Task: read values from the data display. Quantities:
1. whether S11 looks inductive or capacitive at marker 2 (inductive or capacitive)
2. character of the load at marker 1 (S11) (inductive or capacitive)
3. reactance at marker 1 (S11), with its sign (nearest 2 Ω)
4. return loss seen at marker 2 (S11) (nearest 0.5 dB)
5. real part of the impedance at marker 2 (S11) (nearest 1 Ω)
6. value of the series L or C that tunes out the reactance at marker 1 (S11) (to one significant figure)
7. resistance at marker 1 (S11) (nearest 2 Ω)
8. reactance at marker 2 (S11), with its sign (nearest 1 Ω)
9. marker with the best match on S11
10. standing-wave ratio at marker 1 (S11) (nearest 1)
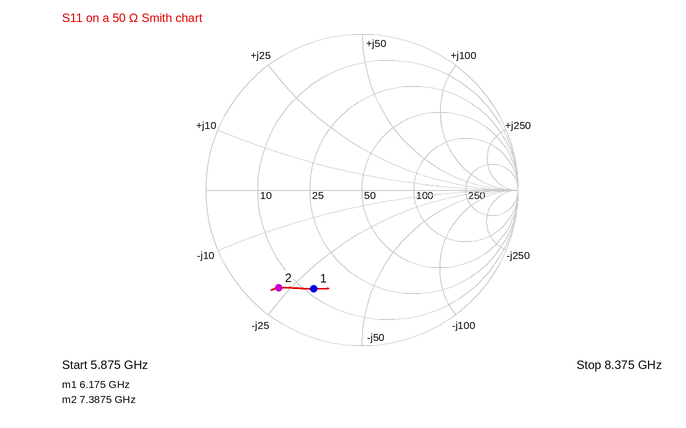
capacitive
capacitive
-30 Ω
1.5 dB
6 Ω
800 pH
12 Ω
-23 Ω
marker 1
6
